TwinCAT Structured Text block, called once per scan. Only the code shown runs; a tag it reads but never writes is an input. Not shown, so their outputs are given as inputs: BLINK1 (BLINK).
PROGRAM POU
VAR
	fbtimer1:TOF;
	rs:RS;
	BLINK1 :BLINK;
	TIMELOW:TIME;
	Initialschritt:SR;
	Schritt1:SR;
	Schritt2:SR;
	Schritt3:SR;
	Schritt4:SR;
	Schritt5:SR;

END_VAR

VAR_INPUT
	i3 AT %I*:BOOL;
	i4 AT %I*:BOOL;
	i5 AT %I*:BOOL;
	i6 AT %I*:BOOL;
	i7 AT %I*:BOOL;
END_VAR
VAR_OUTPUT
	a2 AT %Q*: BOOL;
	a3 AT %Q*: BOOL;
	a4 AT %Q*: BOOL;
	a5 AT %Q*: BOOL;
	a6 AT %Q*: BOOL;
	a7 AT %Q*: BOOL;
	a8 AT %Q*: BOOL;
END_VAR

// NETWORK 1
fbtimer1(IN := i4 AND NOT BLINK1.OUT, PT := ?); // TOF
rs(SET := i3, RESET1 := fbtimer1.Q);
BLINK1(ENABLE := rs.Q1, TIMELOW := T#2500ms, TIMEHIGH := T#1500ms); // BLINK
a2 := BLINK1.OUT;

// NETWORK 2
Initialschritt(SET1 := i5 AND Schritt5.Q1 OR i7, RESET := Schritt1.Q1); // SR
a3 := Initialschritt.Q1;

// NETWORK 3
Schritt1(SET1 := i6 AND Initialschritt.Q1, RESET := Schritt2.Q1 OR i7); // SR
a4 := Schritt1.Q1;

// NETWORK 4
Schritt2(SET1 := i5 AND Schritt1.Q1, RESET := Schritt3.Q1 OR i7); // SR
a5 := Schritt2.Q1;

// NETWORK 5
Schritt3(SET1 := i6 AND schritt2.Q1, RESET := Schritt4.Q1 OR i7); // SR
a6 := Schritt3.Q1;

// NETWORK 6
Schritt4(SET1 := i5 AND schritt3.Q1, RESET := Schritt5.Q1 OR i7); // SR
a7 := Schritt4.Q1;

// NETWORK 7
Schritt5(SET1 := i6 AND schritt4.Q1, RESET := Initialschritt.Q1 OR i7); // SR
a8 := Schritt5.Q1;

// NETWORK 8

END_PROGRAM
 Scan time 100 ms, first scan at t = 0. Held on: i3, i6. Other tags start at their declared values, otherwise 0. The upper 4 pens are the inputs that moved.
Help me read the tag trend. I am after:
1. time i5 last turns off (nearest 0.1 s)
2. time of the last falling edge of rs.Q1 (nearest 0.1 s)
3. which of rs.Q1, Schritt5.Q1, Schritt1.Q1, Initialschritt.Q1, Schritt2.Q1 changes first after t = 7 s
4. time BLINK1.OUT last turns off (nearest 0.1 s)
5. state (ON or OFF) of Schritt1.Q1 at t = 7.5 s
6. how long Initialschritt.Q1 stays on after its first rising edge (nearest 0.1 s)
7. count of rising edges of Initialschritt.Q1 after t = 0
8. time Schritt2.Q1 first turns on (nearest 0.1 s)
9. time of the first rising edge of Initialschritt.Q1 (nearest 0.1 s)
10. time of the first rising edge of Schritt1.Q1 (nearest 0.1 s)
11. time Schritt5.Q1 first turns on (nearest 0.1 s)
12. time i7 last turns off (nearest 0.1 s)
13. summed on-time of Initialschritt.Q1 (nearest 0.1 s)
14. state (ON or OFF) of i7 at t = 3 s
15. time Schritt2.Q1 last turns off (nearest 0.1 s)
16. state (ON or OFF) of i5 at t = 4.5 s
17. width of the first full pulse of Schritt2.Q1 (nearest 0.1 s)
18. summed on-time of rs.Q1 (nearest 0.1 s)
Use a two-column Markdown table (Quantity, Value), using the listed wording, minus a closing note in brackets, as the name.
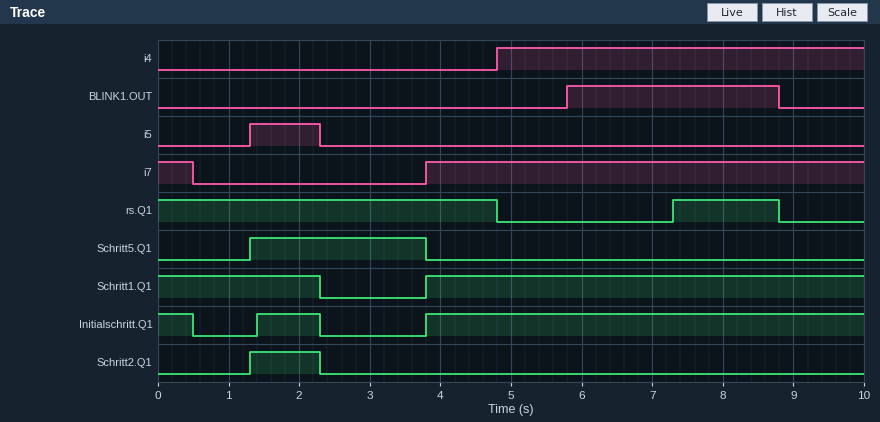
| Quantity | Value |
|---|---|
| time i5 last turns off | 2.3 s |
| time of the last falling edge of rs.Q1 | 8.8 s |
| which of rs.Q1, Schritt5.Q1, Schritt1.Q1, Initialschritt.Q1, Schritt2.Q1 changes first after t = 7 s | rs.Q1 |
| time BLINK1.OUT last turns off | 8.8 s |
| state (ON or OFF) of Schritt1.Q1 at t = 7.5 s | ON |
| how long Initialschritt.Q1 stays on after its first rising edge | 0.9 s |
| count of rising edges of Initialschritt.Q1 after t = 0 | 2 |
| time Schritt2.Q1 first turns on | 1.3 s |
| time of the first rising edge of Initialschritt.Q1 | 1.4 s |
| time of the first rising edge of Schritt1.Q1 | 3.8 s |
| time Schritt5.Q1 first turns on | 1.3 s |
| time i7 last turns off | 0.5 s |
| summed on-time of Initialschritt.Q1 | 7.6 s |
| state (ON or OFF) of i7 at t = 3 s | OFF |
| time Schritt2.Q1 last turns off | 2.3 s |
| state (ON or OFF) of i5 at t = 4.5 s | OFF |
| width of the first full pulse of Schritt2.Q1 | 1.0 s |
| summed on-time of rs.Q1 | 6.3 s |
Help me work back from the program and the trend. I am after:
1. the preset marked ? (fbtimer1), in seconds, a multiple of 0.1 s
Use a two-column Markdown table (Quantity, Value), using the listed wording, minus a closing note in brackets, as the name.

| Quantity | Value |
|---|---|
| the preset marked ? (fbtimer1), in seconds, a multiple of 0.1 s | 1.5 s |
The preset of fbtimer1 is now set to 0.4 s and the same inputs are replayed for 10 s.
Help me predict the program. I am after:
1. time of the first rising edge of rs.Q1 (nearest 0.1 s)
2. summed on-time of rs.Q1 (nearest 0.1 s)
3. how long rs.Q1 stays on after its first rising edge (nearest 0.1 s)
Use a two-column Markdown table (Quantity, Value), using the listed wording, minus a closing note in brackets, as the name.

| Quantity | Value |
|---|---|
| time of the first rising edge of rs.Q1 | 6.2 s |
| summed on-time of rs.Q1 | 7.4 s |
| how long rs.Q1 stays on after its first rising edge | 2.6 s |
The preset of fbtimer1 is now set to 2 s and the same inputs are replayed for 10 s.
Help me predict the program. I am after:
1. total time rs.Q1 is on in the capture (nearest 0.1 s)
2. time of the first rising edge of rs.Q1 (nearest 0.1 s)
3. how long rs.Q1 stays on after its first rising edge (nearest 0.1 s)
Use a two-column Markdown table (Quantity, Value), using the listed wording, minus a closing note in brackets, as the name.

| Quantity | Value |
|---|---|
| total time rs.Q1 is on in the capture | 5.8 s |
| time of the first rising edge of rs.Q1 | 7.8 s |
| how long rs.Q1 stays on after its first rising edge | 1.0 s |
